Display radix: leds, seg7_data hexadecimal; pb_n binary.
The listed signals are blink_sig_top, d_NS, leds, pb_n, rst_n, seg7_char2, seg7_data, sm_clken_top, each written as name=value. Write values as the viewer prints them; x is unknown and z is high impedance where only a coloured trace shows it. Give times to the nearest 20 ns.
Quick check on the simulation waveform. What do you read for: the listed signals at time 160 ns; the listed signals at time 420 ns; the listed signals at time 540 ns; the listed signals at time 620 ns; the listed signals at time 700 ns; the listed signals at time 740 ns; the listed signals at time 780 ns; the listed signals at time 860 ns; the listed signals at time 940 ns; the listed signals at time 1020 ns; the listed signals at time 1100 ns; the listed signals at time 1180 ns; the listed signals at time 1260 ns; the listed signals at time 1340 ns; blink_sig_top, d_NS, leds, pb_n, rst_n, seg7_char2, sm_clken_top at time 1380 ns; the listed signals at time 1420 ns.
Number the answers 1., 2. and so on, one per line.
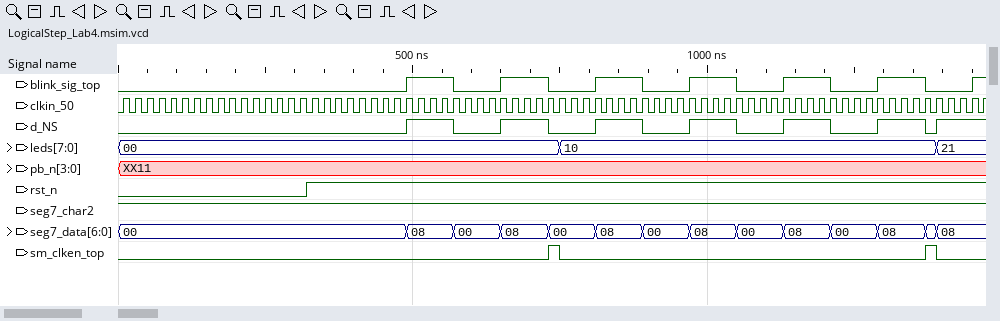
1. blink_sig_top=0, d_NS=0, leds=00, pb_n=XX11, rst_n=0, seg7_char2=1, seg7_data=00, sm_clken_top=0
2. blink_sig_top=0, d_NS=0, leds=00, pb_n=XX11, rst_n=1, seg7_char2=1, seg7_data=00, sm_clken_top=0
3. blink_sig_top=1, d_NS=1, leds=00, pb_n=XX11, rst_n=1, seg7_char2=1, seg7_data=08, sm_clken_top=0
4. blink_sig_top=0, d_NS=0, leds=00, pb_n=XX11, rst_n=1, seg7_char2=1, seg7_data=00, sm_clken_top=0
5. blink_sig_top=1, d_NS=1, leds=00, pb_n=XX11, rst_n=1, seg7_char2=1, seg7_data=08, sm_clken_top=0
6. blink_sig_top=0, d_NS=0, leds=00, pb_n=XX11, rst_n=1, seg7_char2=1, seg7_data=00, sm_clken_top=1
7. blink_sig_top=0, d_NS=0, leds=10, pb_n=XX11, rst_n=1, seg7_char2=1, seg7_data=00, sm_clken_top=0
8. blink_sig_top=1, d_NS=1, leds=10, pb_n=XX11, rst_n=1, seg7_char2=1, seg7_data=08, sm_clken_top=0
9. blink_sig_top=0, d_NS=0, leds=10, pb_n=XX11, rst_n=1, seg7_char2=1, seg7_data=00, sm_clken_top=0
10. blink_sig_top=1, d_NS=1, leds=10, pb_n=XX11, rst_n=1, seg7_char2=1, seg7_data=08, sm_clken_top=0
11. blink_sig_top=0, d_NS=0, leds=10, pb_n=XX11, rst_n=1, seg7_char2=1, seg7_data=00, sm_clken_top=0
12. blink_sig_top=1, d_NS=1, leds=10, pb_n=XX11, rst_n=1, seg7_char2=1, seg7_data=08, sm_clken_top=0
13. blink_sig_top=0, d_NS=0, leds=10, pb_n=XX11, rst_n=1, seg7_char2=1, seg7_data=00, sm_clken_top=0
14. blink_sig_top=1, d_NS=1, leds=10, pb_n=XX11, rst_n=1, seg7_char2=1, seg7_data=08, sm_clken_top=0
15. blink_sig_top=0, d_NS=0, leds=10, pb_n=XX11, rst_n=1, seg7_char2=1, sm_clken_top=1
16. blink_sig_top=0, d_NS=1, leds=21, pb_n=XX11, rst_n=1, seg7_char2=1, seg7_data=08, sm_clken_top=0
